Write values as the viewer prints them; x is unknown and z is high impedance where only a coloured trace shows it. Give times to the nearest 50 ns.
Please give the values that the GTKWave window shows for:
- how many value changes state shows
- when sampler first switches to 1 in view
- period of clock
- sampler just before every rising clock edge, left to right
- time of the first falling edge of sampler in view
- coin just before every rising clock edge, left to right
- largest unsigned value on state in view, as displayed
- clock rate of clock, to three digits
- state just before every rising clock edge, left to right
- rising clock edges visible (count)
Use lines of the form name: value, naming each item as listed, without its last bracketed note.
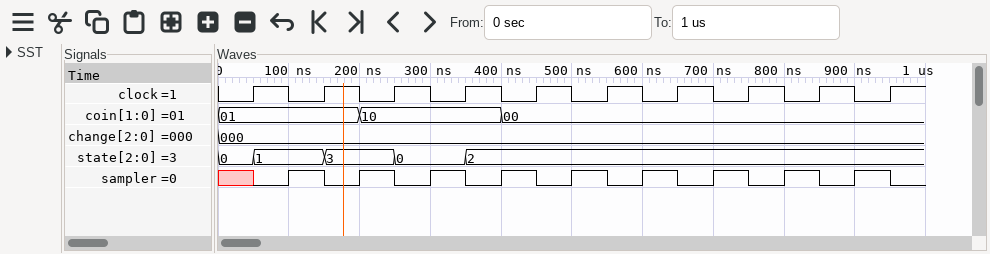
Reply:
how many value changes state shows: 4
when sampler first switches to 1 in view: 100 ns
period of clock: 100 ns
sampler just before every rising clock edge, left to right: x 1 1 1 1 1 1 1 1 1
time of the first falling edge of sampler in view: 150 ns
coin just before every rising clock edge, left to right: 01, 01, 10, 10, 00, 00, 00, 00, 00, 00
largest unsigned value on state in view, as displayed: 3
clock rate of clock, to three digits: 10.0 MHz
state just before every rising clock edge, left to right: 0, 1, 3, 0, 2, 2, 2, 2, 2, 2
rising clock edges visible: 10
